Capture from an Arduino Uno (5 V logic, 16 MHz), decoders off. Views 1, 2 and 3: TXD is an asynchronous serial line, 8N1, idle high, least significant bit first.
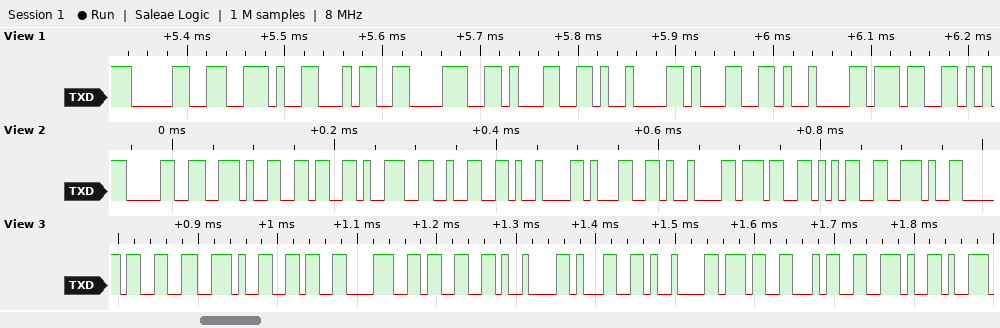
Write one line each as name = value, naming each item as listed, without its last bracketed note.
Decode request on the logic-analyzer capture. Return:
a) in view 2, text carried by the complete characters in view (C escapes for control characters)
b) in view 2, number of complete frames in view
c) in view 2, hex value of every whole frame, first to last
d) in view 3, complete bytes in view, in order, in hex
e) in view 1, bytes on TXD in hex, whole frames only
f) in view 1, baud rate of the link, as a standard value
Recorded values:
in view 2, text carried by the complete characters in view = "0.692\t1\t75."
in view 2, number of complete frames in view = 11
in view 2, hex value of every whole frame, first to last = 30 2E 36 39 32 09 31 09 37 35 2E
in view 3, complete bytes in view, in order, in hex = 33 2E 36 38 33 09 31 09 37 34 2E
in view 1, bytes on TXD in hex, whole frames only = 0x30 0x2E 0x34 0x38 0x31 0x09 0x31 0x09 0x37
in view 1, baud rate of the link, as a standard value = 115200 baud
